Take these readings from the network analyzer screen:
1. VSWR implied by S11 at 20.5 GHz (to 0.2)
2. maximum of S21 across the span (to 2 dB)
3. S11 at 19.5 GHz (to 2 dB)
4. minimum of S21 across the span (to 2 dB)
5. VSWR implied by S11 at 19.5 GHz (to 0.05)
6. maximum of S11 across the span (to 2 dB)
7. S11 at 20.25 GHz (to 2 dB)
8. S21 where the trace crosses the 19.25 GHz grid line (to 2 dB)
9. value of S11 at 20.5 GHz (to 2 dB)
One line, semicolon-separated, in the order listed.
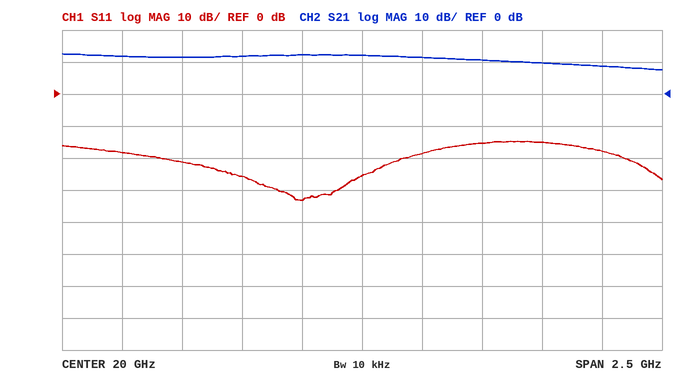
1.4; 12 dB; -26 dB; 8 dB; 1.10; -14 dB; -18 dB; 12 dB; -16 dB
